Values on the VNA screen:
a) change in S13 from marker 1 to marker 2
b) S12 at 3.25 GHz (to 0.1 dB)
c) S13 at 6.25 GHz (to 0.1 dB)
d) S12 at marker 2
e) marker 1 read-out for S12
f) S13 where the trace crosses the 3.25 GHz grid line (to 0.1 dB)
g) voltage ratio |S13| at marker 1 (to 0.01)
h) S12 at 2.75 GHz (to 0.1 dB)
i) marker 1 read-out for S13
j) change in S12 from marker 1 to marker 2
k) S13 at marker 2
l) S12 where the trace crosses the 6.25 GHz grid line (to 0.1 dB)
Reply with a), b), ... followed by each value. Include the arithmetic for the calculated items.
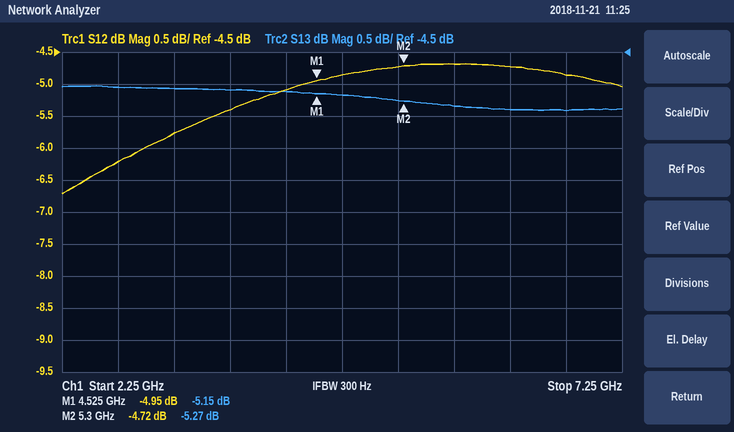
a) -5.27 − (-5.15) = -0.12 dB
b) -5.8 dB
c) -5.4 dB
d) -4.72 dB
e) -4.95 dB
f) -5.1 dB
g) 10^(-5.15/20) ≈ 0.55
h) -6.2 dB
i) -5.15 dB
j) -4.72 − (-4.95) = 0.23 dB
k) -5.27 dB
l) -4.7 dB
